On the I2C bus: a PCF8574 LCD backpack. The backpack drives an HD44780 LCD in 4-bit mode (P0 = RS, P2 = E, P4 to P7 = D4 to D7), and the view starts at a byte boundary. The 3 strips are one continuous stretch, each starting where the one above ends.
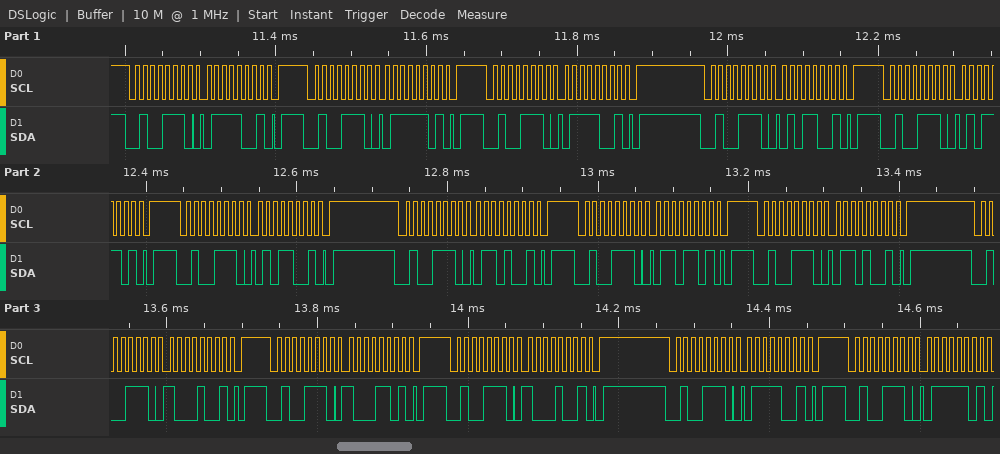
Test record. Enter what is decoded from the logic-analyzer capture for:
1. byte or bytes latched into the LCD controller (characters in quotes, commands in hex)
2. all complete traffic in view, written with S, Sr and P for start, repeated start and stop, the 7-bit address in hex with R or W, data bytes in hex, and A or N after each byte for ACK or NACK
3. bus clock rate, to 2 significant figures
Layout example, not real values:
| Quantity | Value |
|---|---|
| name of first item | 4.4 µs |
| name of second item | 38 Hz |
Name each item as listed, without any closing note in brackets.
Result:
| Quantity | Value |
|---|---|
| byte or bytes latched into the LCD controller | 'u' 'h' |
| all complete traffic in view, written with S, Sr and P for start, repeated start and stop, the 7-bit address in hex with R or W, data bytes in hex, and A or N after each byte for ACK or NACK | S 27W A 79 A P S 27W A 7D A P S 27W A 79 A P S 27W A 59 A P S 27W A 5D A P S 27W A 59 A P S 27W A 69 A P S 27W A 6D A P S 27W A 69 A P S 27W A 89 A P S 27W A 8D A P S 27W A 89 A P S 27W A 79 A P S 27W A 7D A |
| bus clock rate, to 2 significant figures | 100 kHz |
